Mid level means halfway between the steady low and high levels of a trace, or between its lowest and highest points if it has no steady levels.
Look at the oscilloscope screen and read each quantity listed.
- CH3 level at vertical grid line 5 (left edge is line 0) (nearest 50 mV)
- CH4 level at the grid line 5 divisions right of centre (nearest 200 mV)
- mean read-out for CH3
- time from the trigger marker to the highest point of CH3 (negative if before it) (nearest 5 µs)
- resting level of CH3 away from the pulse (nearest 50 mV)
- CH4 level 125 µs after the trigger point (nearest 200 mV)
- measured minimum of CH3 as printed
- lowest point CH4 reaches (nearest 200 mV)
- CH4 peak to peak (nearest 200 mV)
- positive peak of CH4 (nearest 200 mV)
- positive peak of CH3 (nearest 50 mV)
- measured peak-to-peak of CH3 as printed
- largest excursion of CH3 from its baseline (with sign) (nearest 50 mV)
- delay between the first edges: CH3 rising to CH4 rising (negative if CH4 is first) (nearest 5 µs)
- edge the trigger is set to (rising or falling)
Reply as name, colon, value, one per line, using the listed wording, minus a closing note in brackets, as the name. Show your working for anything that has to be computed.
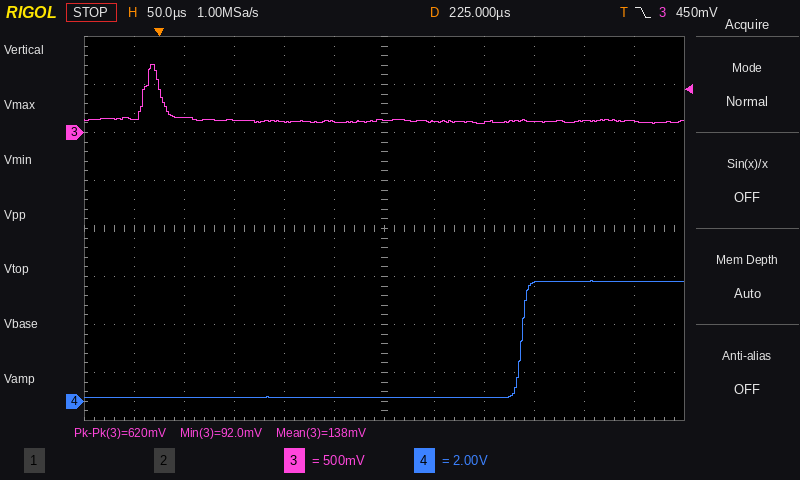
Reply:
CH3 level at vertical grid line 5 (left edge is line 0): 100 mV
CH4 level at the grid line 5 divisions right of centre: 5.0 V
mean read-out for CH3: 138 mV
time from the trigger marker to the highest point of CH3 (negative if before it): -5 µs
resting level of CH3 away from the pulse: 100 mV
CH4 level 125 µs after the trigger point: 200 mV
measured minimum of CH3 as printed: 92.0 mV
lowest point CH4 reaches: 200 mV
CH4 peak to peak: 5.0 V − (200 mV) = 4.8 V
positive peak of CH4: 5.0 V
positive peak of CH3: 700 mV
measured peak-to-peak of CH3 as printed: 620 mV
largest excursion of CH3 from its baseline (with sign): 700 mV − (100 mV) = +600 mV
delay between the first edges: CH3 rising to CH4 rising (negative if CH4 is first): +380 µs
edge the trigger is set to: falling
